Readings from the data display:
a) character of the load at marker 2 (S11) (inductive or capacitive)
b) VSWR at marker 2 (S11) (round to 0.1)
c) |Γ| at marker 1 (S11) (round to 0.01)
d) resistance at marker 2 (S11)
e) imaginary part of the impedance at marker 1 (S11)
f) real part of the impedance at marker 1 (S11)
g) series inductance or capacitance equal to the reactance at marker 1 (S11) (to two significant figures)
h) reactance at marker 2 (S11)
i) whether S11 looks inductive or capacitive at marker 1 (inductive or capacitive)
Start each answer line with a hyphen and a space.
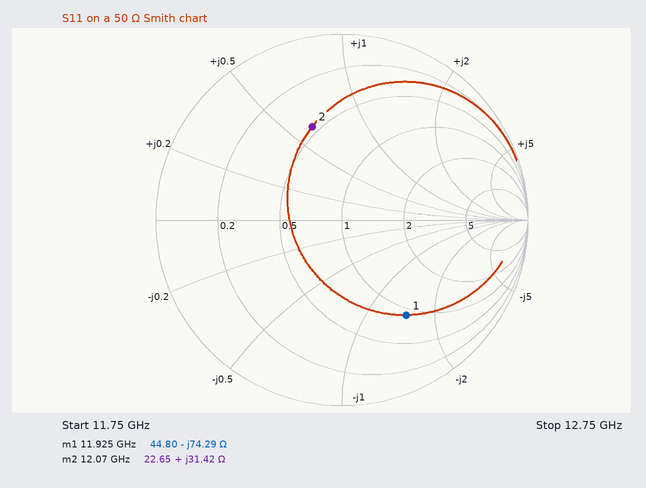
- inductive
- 3.2
- 0.62
- 22.65 Ω
- -74.29 Ω
- 44.80 Ω
- 180 fF
- +31.42 Ω
- capacitive
